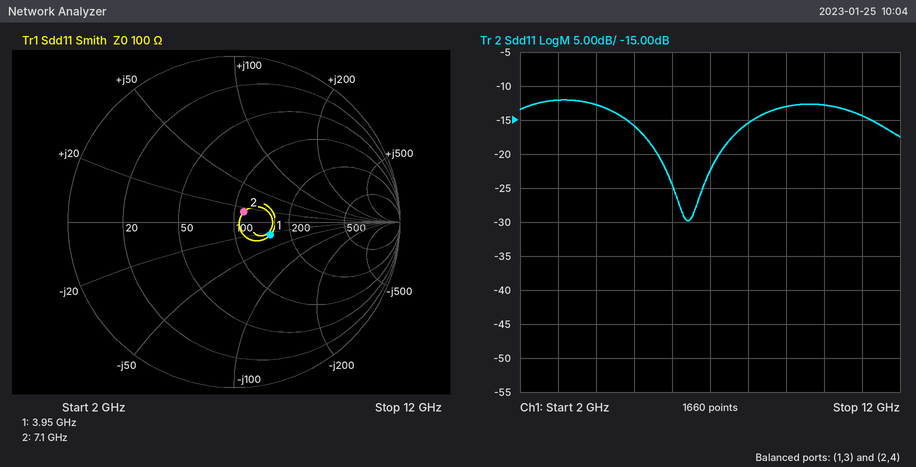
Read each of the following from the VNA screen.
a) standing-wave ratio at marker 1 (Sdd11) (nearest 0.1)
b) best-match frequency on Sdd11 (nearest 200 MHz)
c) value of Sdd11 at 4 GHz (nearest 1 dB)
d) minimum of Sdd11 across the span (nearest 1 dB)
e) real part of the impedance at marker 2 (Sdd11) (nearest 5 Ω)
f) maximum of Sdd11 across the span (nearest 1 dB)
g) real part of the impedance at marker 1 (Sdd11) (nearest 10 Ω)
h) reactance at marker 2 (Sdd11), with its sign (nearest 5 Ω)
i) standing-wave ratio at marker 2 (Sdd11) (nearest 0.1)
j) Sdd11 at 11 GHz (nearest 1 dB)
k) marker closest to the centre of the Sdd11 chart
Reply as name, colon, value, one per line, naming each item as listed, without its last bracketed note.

standing-wave ratio at marker 1 (Sdd11): 1.6
best-match frequency on Sdd11: 6.4 GHz
value of Sdd11 at 4 GHz: -13 dB
minimum of Sdd11 across the span: -30 dB
real part of the impedance at marker 2 (Sdd11): 110 Ω
maximum of Sdd11 across the span: -12 dB
real part of the impedance at marker 1 (Sdd11): 150 Ω
reactance at marker 2 (Sdd11), with its sign: +15 Ω
standing-wave ratio at marker 2 (Sdd11): 1.2
Sdd11 at 11 GHz: -14 dB
marker closest to the centre of the Sdd11 chart: marker 2
